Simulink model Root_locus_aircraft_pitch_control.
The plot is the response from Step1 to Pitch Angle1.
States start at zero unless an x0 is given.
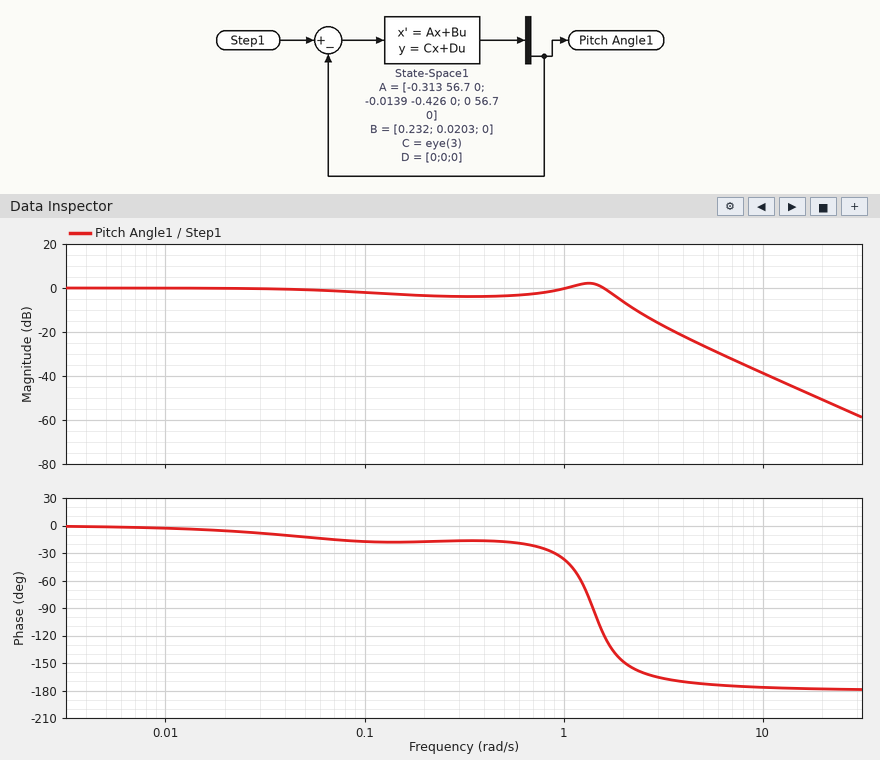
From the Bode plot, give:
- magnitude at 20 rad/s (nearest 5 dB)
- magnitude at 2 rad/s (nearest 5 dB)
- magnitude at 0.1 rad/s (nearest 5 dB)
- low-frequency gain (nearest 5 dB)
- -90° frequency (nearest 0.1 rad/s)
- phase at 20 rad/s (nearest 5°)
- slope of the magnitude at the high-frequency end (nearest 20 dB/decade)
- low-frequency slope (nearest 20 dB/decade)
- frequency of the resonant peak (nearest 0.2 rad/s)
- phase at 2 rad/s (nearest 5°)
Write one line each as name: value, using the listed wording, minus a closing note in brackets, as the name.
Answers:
magnitude at 20 rad/s: -50 dB
magnitude at 2 rad/s: -5 dB
magnitude at 0.1 rad/s: 0 dB
low-frequency gain: 0 dB
-90° frequency: 1.4 rad/s
phase at 20 rad/s: -180°
slope of the magnitude at the high-frequency end: -40 dB/decade
low-frequency slope: 0 dB/decade
frequency of the resonant peak: 1.4 rad/s
phase at 2 rad/s: -150°
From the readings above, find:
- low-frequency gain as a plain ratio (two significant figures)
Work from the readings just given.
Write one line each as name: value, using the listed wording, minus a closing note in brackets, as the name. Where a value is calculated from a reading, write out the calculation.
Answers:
low-frequency gain as a plain ratio: 10^(0 / 20) = 1.0
